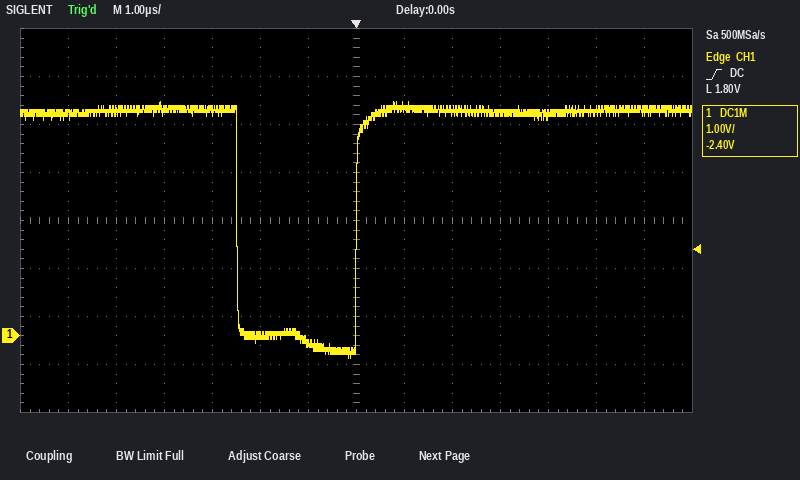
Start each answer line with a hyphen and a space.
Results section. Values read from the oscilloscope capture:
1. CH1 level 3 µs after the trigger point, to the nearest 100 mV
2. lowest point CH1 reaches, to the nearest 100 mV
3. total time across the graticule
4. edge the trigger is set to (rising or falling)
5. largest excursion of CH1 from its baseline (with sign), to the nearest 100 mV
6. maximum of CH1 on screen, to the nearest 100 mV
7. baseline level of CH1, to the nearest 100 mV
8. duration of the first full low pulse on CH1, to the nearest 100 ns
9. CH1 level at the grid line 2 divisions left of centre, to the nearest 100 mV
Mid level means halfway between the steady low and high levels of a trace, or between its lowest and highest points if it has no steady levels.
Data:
- 4.6 V
- -500 mV
- 14 µs
- rising
- -5.2 V
- 4.9 V
- 4.7 V
- 2.5 µs
- 0.0 V
